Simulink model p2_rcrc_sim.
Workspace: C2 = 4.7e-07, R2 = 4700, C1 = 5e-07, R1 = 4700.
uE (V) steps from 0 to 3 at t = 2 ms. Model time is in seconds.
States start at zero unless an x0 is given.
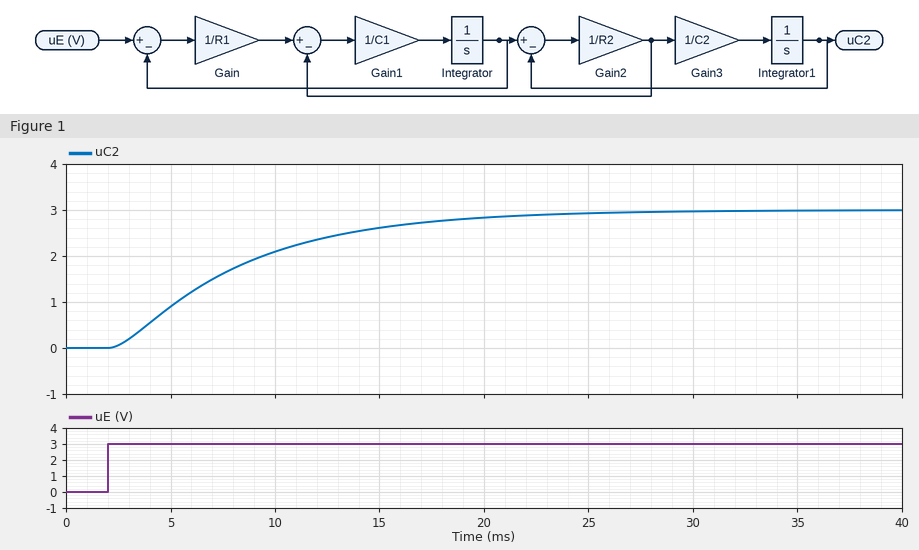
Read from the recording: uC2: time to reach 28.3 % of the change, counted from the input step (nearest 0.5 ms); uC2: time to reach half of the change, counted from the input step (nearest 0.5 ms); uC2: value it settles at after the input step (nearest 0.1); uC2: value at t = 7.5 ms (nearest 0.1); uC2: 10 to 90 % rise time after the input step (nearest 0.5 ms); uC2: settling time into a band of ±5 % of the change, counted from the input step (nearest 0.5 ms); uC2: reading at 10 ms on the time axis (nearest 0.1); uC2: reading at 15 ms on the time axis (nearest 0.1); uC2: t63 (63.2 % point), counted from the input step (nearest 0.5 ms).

3.0 ms
5.0 ms
3.0
1.6
13.0 ms
18.5 ms
2.1
2.6
7.0 ms
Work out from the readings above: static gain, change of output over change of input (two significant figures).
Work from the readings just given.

1.0
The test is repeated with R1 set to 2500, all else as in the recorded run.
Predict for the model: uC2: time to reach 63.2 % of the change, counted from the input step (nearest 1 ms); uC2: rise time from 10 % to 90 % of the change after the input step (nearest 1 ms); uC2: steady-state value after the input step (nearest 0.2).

5 ms
9 ms
3.0
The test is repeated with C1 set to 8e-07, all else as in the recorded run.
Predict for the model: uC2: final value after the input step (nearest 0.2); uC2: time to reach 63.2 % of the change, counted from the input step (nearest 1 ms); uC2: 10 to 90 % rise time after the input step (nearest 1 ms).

3.0
8 ms
16 ms
